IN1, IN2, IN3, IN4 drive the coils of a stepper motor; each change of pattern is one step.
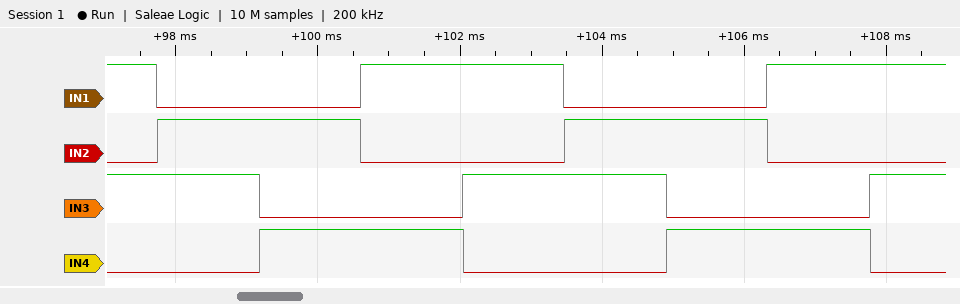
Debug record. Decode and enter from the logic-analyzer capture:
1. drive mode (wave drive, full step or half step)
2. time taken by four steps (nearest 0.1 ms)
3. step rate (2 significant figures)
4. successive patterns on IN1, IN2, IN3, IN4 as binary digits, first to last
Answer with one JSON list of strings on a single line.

["full step", "5.7 ms", "700 steps/s", "1010 0110 0101 1001 1010 0110 0101 1001 1010"]
